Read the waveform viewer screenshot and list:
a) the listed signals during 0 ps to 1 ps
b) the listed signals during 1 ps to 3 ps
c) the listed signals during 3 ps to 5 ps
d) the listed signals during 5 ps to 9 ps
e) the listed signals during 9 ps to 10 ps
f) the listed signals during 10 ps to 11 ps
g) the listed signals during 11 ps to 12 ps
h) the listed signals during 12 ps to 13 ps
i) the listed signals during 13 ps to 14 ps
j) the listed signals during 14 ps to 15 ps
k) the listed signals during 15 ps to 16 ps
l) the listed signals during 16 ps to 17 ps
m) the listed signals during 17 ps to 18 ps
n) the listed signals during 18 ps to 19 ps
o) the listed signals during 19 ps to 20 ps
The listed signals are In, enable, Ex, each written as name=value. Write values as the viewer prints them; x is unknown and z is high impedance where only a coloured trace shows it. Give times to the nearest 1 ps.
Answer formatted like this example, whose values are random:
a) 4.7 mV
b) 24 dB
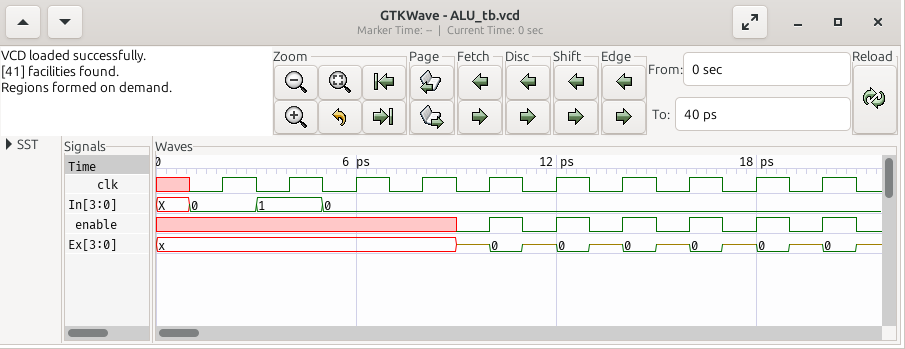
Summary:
a) In=X, enable=x, Ex=x
b) In=0, enable=x, Ex=x
c) In=1, enable=x, Ex=x
d) In=0, enable=x, Ex=x
e) In=0, enable=0, Ex=z
f) In=0, enable=1, Ex=0
g) In=0, enable=0, Ex=z
h) In=0, enable=1, Ex=0
i) In=0, enable=0, Ex=z
j) In=0, enable=1, Ex=0
k) In=0, enable=0, Ex=z
l) In=0, enable=1, Ex=0
m) In=0, enable=0, Ex=z
n) In=0, enable=1, Ex=0
o) In=0, enable=0, Ex=z
